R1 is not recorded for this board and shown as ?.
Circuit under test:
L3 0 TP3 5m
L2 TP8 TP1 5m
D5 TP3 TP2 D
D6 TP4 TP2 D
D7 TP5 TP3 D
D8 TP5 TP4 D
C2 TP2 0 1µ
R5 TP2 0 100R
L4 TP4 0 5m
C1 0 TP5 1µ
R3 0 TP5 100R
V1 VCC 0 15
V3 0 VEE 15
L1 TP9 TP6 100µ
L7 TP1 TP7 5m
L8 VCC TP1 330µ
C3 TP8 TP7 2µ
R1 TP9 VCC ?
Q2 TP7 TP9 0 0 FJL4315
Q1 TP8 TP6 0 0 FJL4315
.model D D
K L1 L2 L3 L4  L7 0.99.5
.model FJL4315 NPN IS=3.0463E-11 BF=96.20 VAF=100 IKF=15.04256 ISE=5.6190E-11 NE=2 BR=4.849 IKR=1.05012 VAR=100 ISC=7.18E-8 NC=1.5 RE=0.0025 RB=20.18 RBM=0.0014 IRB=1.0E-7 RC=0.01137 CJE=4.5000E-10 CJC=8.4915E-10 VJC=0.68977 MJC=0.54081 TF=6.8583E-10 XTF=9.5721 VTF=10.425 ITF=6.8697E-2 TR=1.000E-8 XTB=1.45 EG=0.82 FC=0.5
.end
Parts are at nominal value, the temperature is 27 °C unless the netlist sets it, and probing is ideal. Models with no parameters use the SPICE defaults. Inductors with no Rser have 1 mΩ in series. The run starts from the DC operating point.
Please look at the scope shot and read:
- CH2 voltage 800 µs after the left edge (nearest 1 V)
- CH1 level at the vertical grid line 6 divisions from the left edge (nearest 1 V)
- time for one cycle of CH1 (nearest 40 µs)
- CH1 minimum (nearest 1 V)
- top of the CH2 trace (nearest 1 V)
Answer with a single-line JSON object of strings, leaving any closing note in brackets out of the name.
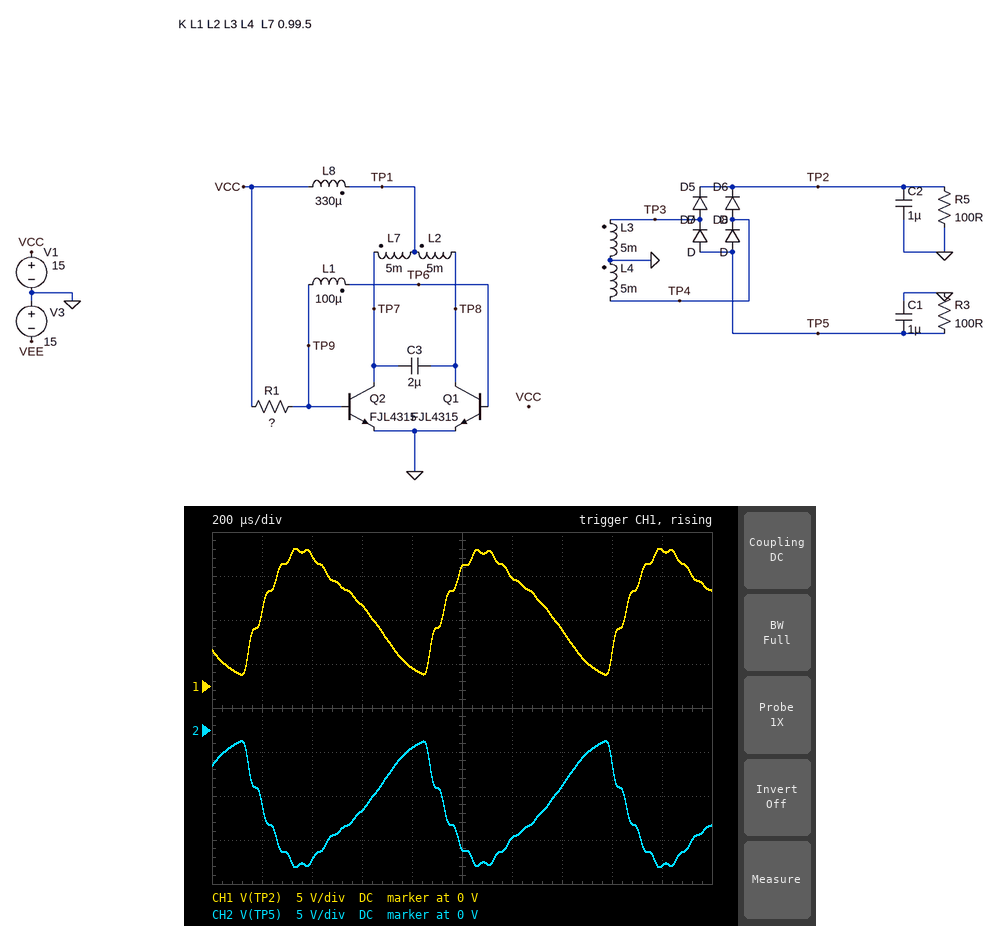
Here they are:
{"CH2 voltage 800 µs after the left edge": "-2 V", "CH1 level at the vertical grid line 6 divisions from the left edge": "12 V", "time for one cycle of CH1": "720 µs", "CH1 minimum": "1 V", "top of the CH2 trace": "-1 V"}
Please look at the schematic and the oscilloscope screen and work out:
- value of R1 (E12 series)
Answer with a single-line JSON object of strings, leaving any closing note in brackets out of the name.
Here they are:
{"value of R1": "4.7 kΩ"}
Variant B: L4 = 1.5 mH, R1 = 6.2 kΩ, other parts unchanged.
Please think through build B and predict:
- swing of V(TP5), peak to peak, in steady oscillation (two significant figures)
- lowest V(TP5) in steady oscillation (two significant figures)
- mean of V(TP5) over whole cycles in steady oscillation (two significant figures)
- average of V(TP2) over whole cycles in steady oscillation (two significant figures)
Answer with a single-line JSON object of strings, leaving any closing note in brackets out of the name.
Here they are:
{"swing of V(TP5), peak to peak, in steady oscillation": "15 V", "lowest V(TP5) in steady oscillation": "-16 V", "mean of V(TP5) over whole cycles in steady oscillation": "-7.2 V", "average of V(TP2) over whole cycles in steady oscillation": "7.2 V"}
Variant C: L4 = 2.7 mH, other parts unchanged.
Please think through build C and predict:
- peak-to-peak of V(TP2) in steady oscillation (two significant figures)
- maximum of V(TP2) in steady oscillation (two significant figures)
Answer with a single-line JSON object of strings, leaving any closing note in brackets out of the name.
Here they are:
{"peak-to-peak of V(TP2) in steady oscillation": "16 V", "maximum of V(TP2) in steady oscillation": "17 V"}
